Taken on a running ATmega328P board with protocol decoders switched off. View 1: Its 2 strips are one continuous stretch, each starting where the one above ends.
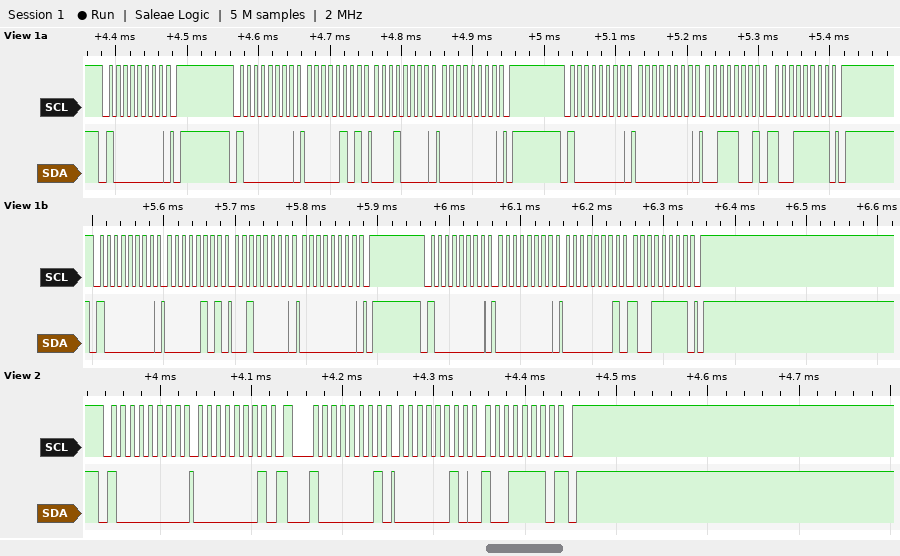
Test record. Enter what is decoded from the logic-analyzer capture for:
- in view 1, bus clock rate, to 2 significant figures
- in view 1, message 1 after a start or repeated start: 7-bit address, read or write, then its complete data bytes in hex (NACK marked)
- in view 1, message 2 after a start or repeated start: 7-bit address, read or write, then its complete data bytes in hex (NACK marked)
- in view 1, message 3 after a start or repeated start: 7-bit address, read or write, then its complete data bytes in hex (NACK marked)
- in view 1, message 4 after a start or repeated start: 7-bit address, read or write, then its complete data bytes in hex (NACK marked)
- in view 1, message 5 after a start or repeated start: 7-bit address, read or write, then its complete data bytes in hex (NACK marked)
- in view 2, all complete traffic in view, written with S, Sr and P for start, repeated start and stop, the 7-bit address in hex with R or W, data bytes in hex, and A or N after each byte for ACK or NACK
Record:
100 kHz
0x40 write
0x40 write: 05 10 00
0x40 write: 00 39 9F
0x40 write: 05 20 00
0x40 write: 00 01 9F
S 40W A 01 A Sr 40R A 02 A 9E N P
